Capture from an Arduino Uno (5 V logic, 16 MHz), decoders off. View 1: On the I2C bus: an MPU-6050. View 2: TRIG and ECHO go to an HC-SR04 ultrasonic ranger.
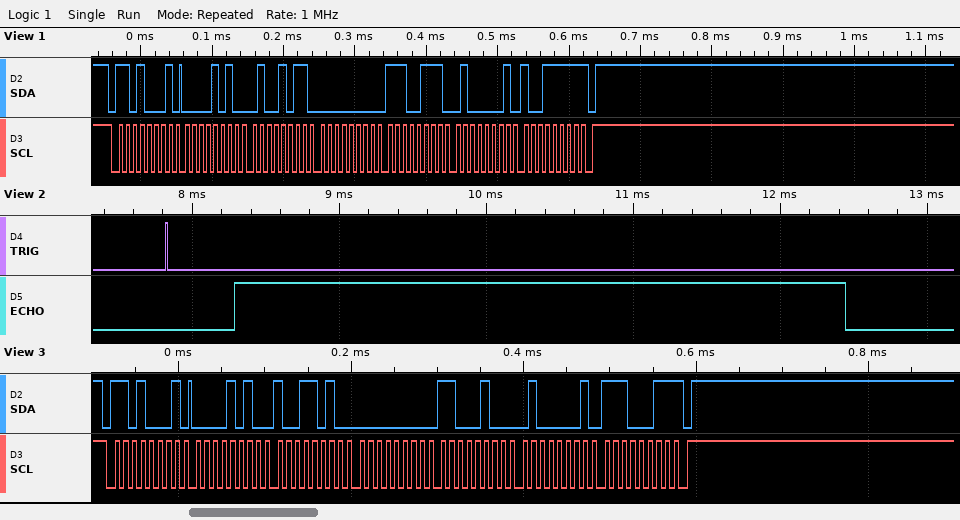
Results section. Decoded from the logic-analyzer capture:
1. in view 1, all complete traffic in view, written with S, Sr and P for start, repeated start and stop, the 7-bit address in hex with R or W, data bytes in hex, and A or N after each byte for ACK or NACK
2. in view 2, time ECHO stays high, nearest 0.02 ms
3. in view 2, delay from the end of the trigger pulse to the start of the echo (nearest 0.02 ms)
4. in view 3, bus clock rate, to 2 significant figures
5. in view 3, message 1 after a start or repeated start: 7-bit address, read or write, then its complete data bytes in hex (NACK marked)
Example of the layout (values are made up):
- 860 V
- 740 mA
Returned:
- S 68R A 0A A 4B A 00 A E7 A 41 A 9F N P
- 4.16 ms
- 0.46 ms
- 100 kHz
- 0x68 read: 0A 9A 00 C4 41 E3 NACK
